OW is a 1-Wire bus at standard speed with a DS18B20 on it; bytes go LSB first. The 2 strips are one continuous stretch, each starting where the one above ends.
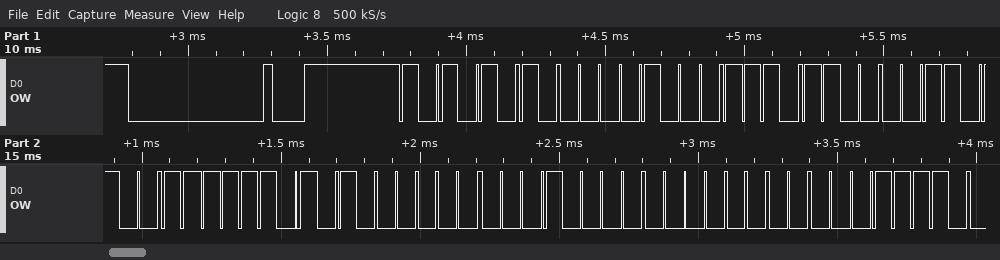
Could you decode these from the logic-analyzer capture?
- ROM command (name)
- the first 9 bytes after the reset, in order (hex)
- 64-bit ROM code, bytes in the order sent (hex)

Match ROM
55 10 37 2C BF 02 08 00 78
10 37 2C BF 02 08 00 78
